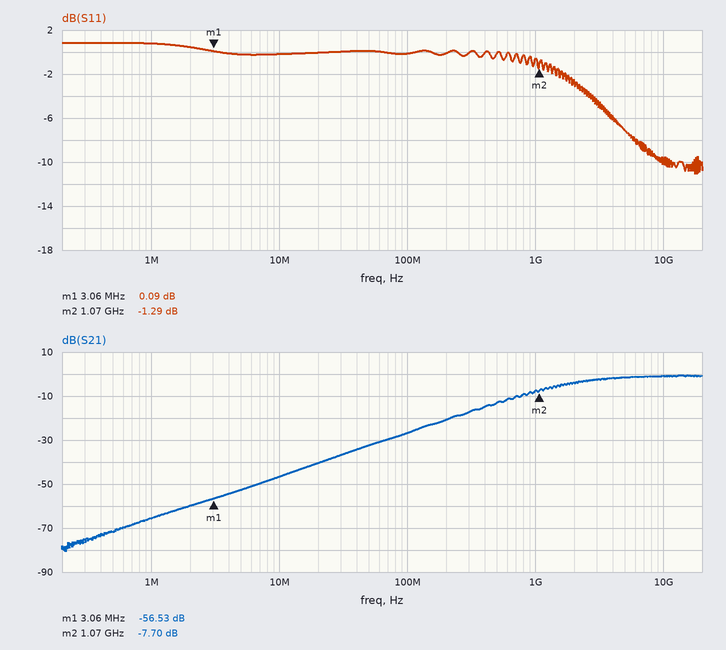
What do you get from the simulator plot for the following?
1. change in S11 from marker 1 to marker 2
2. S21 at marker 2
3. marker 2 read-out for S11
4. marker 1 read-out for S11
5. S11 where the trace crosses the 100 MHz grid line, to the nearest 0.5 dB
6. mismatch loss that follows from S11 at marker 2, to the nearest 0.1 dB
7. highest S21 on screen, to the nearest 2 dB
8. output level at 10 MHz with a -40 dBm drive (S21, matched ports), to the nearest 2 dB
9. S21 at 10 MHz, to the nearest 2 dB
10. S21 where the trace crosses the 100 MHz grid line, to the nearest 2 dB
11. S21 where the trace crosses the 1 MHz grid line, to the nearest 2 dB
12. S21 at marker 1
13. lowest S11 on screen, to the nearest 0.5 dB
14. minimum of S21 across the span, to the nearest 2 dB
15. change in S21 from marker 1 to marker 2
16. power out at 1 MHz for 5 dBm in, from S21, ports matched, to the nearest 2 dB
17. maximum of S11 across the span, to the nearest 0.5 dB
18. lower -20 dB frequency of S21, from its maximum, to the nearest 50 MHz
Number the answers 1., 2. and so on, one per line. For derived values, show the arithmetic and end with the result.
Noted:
1. -1.29 − (0.09) = -1.38 dB
2. -7.70 dB
3. -1.29 dB
4. 0.09 dB
5. 0.0 dB
6. −10 log10(1 − 10^(-1.29/10)) ≈ 5.9 dB
7. 0 dB
8. -40 dBm + (-46 dB) = -86 dBm
9. -46 dB
10. -26 dB
11. -66 dB
12. -56.53 dB
13. -11.0 dB
14. -80 dB
15. -7.7 − (-56.53) = 48.83 dB
16. 5 dBm + (-66 dB) = -60 dBm
17. 1.0 dB
18. 200 MHz
